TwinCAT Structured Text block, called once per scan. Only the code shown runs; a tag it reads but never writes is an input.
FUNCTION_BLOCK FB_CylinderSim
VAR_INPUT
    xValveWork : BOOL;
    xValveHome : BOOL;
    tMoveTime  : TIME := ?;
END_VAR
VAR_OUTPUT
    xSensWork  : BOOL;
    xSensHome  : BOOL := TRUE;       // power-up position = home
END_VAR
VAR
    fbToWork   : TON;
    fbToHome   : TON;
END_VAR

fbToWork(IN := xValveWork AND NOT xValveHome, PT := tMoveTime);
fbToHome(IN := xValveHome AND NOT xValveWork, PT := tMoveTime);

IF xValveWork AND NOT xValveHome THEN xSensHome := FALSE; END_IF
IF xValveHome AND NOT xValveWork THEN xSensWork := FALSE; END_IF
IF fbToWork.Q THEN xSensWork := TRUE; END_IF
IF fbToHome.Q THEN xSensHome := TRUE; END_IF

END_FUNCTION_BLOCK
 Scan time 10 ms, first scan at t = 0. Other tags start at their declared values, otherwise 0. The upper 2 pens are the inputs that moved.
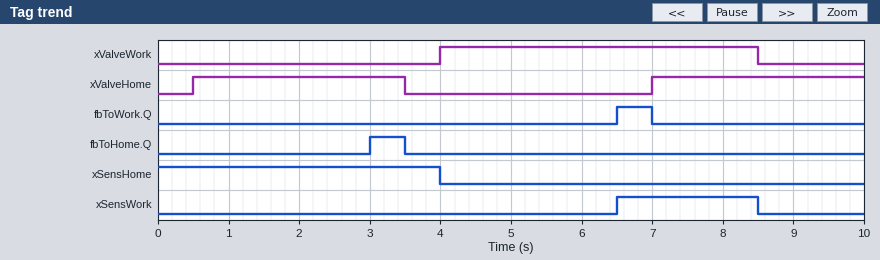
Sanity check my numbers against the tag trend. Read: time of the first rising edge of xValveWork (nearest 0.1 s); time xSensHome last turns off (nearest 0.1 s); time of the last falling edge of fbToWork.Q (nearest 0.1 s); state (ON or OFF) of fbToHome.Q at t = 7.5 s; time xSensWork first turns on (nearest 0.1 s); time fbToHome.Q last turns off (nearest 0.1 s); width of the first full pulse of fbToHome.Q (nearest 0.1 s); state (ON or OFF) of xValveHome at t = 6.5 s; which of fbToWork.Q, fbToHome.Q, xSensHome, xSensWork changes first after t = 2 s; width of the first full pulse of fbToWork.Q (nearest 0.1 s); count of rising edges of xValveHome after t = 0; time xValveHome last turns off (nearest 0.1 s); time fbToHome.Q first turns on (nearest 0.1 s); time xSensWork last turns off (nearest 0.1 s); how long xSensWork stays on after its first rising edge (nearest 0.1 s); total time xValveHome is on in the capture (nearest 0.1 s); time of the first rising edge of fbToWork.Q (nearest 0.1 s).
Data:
4.0 s
4.0 s
7.0 s
OFF
6.5 s
3.5 s
0.5 s
OFF
fbToHome.Q
0.5 s
2
3.5 s
3.0 s
8.5 s
2.0 s
6.0 s
6.5 s
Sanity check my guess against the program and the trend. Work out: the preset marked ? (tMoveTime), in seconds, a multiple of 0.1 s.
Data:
2.5 s
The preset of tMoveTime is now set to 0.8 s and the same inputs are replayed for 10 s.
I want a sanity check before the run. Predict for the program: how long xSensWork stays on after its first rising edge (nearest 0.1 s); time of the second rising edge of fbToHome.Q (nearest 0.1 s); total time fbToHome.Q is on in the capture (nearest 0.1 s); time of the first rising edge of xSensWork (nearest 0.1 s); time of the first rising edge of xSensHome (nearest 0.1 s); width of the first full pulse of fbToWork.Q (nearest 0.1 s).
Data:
3.7 s
9.3 s
2.9 s
4.8 s
9.3 s
2.2 s
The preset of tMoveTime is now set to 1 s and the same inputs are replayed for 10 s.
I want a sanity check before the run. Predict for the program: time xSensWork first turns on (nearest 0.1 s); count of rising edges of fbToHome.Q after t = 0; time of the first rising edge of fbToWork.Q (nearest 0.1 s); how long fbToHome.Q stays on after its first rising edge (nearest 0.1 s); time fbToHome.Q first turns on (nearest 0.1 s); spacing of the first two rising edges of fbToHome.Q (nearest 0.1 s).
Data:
5.0 s
2
5.0 s
2.0 s
1.5 s
8.0 s
